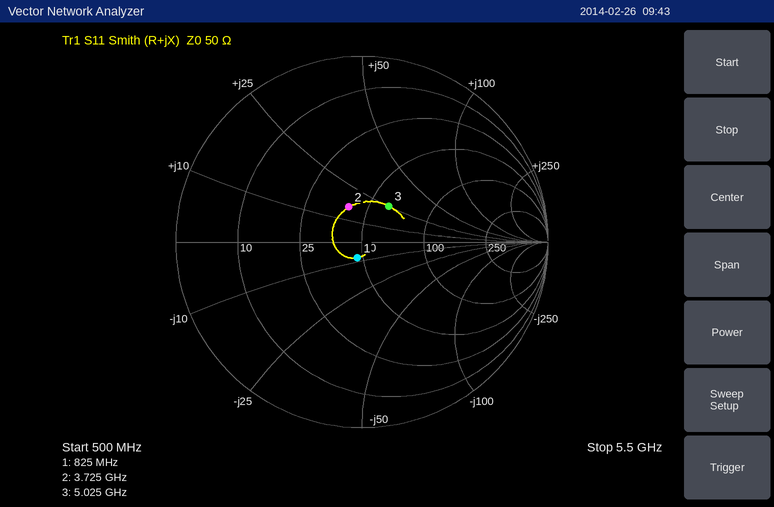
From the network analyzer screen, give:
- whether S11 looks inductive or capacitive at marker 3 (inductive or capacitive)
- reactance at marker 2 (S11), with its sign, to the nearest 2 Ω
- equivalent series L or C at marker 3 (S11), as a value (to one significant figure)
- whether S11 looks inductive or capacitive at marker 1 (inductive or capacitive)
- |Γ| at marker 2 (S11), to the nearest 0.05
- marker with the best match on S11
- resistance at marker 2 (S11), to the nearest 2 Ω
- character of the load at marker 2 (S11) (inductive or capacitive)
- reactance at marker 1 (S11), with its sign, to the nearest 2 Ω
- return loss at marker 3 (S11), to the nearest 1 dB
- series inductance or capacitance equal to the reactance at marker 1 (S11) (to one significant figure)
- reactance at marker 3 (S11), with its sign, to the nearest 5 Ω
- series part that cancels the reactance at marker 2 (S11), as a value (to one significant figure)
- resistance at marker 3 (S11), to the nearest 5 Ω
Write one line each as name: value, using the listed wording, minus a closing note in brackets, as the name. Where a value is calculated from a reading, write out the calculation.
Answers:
whether S11 looks inductive or capacitive at marker 3: inductive
reactance at marker 2 (S11), with its sign, to the nearest 2 Ω: +16 Ω
equivalent series L or C at marker 3 (S11), as a value: L = 25 Ω/(2π × 5.025 GHz) ≈ 792 pH, so 800 pH to one significant figure
whether S11 looks inductive or capacitive at marker 1: capacitive
|Γ| at marker 2 (S11), to the nearest 0.05: 0.20
marker with the best match on S11: marker 1
resistance at marker 2 (S11), to the nearest 2 Ω: 40 Ω
character of the load at marker 2 (S11): inductive
reactance at marker 1 (S11), with its sign, to the nearest 2 Ω: -8 Ω
return loss at marker 3 (S11), to the nearest 1 dB: 12 dB
series inductance or capacitance equal to the reactance at marker 1 (S11): C = 1/(2π × 825 MHz × 8 Ω) ≈ 24.1 pF, so 20 pF to one significant figure
reactance at marker 3 (S11), with its sign, to the nearest 5 Ω: +25 Ω
series part that cancels the reactance at marker 2 (S11), as a value: C = 1/(2π × 3.725 GHz × 16 Ω) ≈ 3 pF
resistance at marker 3 (S11), to the nearest 5 Ω: 60 Ω
